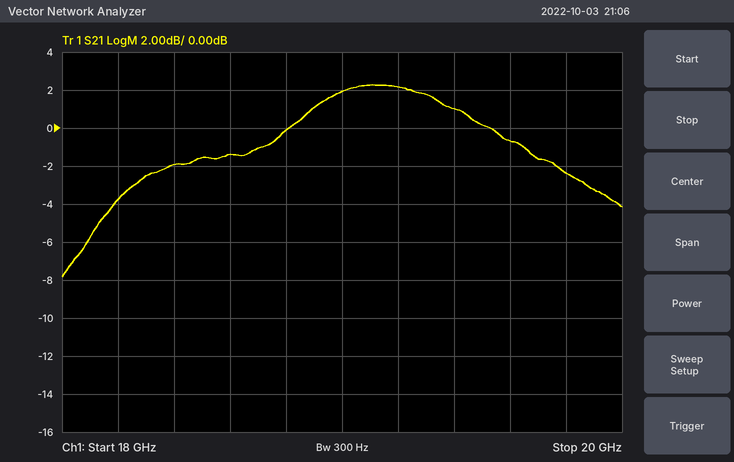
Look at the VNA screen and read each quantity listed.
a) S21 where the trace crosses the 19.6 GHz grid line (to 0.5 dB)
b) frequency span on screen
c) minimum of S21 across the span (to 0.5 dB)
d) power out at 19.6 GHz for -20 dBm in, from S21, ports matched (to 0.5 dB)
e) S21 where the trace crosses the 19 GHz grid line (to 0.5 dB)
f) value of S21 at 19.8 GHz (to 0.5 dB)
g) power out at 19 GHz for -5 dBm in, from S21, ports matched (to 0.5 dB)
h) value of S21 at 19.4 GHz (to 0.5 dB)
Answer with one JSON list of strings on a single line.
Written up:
["-0.5 dB", "2 GHz", "-8.0 dB", "-20.5 dBm", "2.0 dB", "-2.5 dB", "-3.0 dBm", "1.0 dB"]
